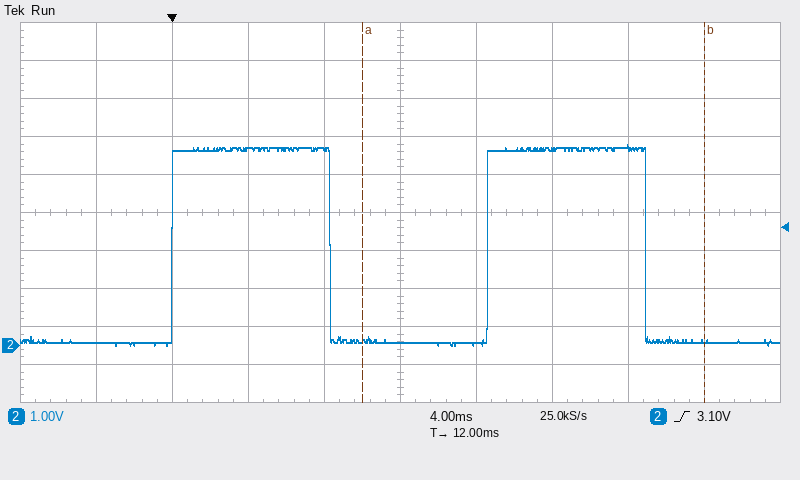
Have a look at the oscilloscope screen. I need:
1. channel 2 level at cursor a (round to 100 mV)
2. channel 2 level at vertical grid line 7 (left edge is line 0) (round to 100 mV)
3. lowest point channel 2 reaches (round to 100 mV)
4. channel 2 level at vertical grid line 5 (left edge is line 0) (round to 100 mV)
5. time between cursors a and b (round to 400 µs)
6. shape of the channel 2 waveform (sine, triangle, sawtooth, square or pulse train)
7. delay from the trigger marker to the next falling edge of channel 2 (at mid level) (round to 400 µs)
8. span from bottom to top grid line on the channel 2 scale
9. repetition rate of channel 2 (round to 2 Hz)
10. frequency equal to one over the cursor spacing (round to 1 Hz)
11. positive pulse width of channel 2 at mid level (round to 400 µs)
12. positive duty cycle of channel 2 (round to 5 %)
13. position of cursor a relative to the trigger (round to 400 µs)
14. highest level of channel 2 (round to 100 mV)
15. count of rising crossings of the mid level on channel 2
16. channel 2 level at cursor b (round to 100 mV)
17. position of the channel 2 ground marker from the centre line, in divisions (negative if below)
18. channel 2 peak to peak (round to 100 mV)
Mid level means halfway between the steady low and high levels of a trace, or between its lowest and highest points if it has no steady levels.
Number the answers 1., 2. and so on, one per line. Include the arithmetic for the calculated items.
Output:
1. 100 mV
2. 5.2 V
3. 0.0 V
4. 100 mV
5. 18.0 ms
6. square
7. 8.4 ms
8. 10 V
9. 60 Hz
10. 1 / 18.0 ms ≈ 56 Hz
11. 8.4 ms
12. 50 %
13. +10.0 ms
14. 5.3 V
15. 2
16. 100 mV
17. -3.5 div
18. 5.3 V − (0.0 V) = 5.3 V
